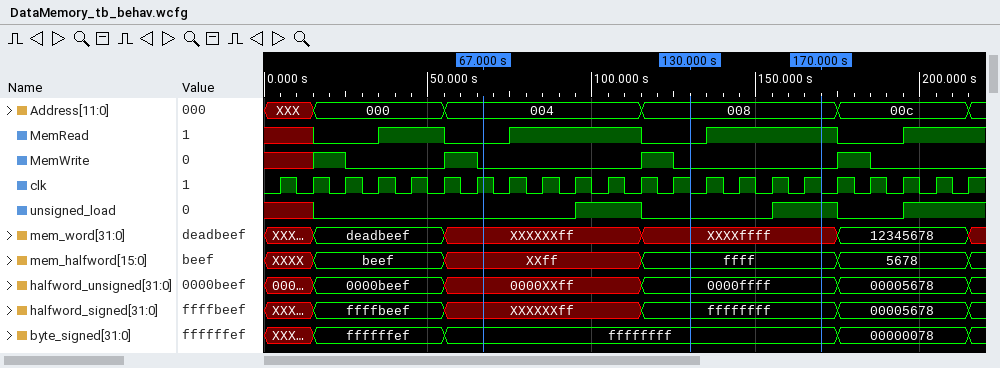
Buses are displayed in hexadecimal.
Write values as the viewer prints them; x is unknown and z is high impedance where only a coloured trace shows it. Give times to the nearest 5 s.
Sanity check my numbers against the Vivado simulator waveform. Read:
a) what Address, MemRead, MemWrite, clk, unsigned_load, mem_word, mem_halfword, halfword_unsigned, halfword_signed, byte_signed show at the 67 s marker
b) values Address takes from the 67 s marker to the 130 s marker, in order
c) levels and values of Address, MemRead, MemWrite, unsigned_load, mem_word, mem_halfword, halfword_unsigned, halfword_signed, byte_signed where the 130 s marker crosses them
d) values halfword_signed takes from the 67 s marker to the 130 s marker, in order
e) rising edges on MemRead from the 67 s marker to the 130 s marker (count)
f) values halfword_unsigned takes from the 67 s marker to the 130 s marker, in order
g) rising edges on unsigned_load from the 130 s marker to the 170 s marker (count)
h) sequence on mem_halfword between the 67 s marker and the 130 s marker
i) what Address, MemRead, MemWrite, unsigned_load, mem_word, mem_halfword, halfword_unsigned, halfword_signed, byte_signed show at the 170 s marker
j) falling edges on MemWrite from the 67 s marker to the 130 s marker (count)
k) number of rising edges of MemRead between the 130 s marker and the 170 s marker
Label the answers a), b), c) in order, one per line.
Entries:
a) Address=004, MemRead=0, MemWrite=0, clk=1, unsigned_load=0, mem_word=XXXXXXff, mem_halfword=XXff, halfword_unsigned=0000XXff, halfword_signed=XXXXXXff, byte_signed=ffffffff
b) 004, 008
c) Address=008, MemRead=0, MemWrite=0, unsigned_load=0, mem_word=XXXXffff, mem_halfword=ffff, halfword_unsigned=0000ffff, halfword_signed=ffffffff, byte_signed=ffffffff
d) XXXXXXff, ffffffff
e) 1
f) 0000XXff, 0000ffff
g) 1
h) XXff, ffff
i) Address=008, MemRead=1, MemWrite=0, unsigned_load=1, mem_word=XXXXffff, mem_halfword=ffff, halfword_unsigned=0000ffff, halfword_signed=ffffffff, byte_signed=ffffffff
j) 1
k) 1
